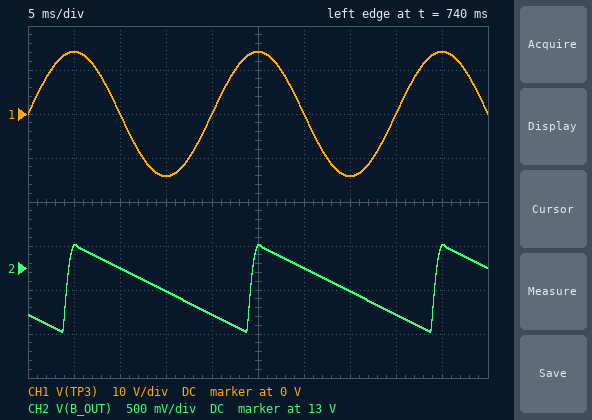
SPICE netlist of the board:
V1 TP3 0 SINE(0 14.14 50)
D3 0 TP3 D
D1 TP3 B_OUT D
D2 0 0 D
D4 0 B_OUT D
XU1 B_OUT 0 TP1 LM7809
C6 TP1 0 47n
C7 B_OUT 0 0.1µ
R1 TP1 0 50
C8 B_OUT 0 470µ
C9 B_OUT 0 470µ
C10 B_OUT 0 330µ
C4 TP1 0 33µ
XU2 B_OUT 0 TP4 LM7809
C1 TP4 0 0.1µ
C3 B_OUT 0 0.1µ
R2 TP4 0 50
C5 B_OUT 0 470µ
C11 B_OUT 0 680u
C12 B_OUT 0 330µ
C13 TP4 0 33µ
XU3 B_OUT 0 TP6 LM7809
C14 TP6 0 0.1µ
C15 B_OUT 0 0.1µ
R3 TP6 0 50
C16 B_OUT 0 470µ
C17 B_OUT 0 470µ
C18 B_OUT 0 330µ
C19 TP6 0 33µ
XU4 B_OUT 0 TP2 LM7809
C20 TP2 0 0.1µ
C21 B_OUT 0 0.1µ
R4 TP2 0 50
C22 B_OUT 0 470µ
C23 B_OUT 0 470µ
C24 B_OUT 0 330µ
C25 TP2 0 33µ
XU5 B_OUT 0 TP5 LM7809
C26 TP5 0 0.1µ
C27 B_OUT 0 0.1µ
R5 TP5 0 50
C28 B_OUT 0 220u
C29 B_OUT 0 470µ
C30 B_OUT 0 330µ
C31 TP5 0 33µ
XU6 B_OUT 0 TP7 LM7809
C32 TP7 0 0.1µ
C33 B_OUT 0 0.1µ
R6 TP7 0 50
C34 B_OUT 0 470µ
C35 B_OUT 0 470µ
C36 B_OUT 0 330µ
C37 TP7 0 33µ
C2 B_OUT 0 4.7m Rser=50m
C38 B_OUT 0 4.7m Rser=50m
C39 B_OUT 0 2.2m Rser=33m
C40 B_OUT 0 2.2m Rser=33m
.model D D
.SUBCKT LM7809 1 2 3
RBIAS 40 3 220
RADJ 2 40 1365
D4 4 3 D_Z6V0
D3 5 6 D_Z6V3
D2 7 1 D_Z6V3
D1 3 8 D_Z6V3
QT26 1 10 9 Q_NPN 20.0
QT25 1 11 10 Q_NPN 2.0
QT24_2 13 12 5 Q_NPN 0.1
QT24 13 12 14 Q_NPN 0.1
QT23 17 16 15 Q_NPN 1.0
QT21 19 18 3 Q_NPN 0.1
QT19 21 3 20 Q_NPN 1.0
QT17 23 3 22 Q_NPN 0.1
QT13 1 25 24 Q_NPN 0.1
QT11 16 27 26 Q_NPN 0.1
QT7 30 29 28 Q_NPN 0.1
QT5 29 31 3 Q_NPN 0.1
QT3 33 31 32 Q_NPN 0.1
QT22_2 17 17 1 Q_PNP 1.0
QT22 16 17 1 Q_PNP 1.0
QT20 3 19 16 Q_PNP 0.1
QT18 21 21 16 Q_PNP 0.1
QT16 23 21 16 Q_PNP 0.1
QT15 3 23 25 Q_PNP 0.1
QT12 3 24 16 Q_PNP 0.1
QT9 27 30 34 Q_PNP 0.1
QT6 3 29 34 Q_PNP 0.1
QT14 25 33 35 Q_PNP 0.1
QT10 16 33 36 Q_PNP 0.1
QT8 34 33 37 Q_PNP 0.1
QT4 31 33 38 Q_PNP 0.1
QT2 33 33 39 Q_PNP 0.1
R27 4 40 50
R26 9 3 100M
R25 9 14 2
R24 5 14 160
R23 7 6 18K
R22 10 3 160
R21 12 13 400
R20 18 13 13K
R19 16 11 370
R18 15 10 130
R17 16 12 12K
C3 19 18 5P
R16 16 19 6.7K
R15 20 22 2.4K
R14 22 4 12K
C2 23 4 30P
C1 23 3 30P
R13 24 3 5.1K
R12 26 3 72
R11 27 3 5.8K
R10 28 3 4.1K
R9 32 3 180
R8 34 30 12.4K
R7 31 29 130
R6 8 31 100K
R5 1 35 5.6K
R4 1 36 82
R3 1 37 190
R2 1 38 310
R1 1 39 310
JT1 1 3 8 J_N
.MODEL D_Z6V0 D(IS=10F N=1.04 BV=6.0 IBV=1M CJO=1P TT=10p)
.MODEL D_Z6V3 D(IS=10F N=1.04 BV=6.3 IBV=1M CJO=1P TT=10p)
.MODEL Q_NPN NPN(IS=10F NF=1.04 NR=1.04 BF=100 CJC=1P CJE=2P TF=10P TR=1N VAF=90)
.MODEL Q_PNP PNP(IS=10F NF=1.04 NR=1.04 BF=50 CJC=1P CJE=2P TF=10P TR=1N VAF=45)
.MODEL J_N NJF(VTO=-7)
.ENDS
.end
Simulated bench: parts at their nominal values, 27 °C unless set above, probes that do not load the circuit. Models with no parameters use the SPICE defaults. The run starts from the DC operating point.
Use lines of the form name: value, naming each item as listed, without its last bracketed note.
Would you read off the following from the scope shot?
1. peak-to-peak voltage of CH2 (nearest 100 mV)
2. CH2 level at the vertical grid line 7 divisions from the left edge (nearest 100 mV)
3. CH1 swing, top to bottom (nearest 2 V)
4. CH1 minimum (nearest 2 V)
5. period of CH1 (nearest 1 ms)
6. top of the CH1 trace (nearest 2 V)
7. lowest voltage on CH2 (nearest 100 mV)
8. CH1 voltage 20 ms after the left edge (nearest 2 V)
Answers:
peak-to-peak voltage of CH2: 1.0 V
CH2 level at the vertical grid line 7 divisions from the left edge: 12.7 V
CH1 swing, top to bottom: 28 V
CH1 minimum: -14 V
period of CH1: 20 ms
top of the CH1 trace: 14 V
lowest voltage on CH2: 12.3 V
CH1 voltage 20 ms after the left edge: 0 V
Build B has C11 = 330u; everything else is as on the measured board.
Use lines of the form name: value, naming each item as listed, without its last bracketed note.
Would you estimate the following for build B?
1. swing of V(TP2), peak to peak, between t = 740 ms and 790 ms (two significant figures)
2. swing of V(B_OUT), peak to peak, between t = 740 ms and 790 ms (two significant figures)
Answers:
swing of V(TP2), peak to peak, between t = 740 ms and 790 ms: 4.3 mV
swing of V(B_OUT), peak to peak, between t = 740 ms and 790 ms: 1.0 V
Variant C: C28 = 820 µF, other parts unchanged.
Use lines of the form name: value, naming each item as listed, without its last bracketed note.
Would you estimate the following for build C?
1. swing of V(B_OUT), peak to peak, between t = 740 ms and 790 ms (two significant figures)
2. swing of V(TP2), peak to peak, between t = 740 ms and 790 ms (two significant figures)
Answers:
swing of V(B_OUT), peak to peak, between t = 740 ms and 790 ms: 960 mV
swing of V(TP2), peak to peak, between t = 740 ms and 790 ms: 4.1 mV
